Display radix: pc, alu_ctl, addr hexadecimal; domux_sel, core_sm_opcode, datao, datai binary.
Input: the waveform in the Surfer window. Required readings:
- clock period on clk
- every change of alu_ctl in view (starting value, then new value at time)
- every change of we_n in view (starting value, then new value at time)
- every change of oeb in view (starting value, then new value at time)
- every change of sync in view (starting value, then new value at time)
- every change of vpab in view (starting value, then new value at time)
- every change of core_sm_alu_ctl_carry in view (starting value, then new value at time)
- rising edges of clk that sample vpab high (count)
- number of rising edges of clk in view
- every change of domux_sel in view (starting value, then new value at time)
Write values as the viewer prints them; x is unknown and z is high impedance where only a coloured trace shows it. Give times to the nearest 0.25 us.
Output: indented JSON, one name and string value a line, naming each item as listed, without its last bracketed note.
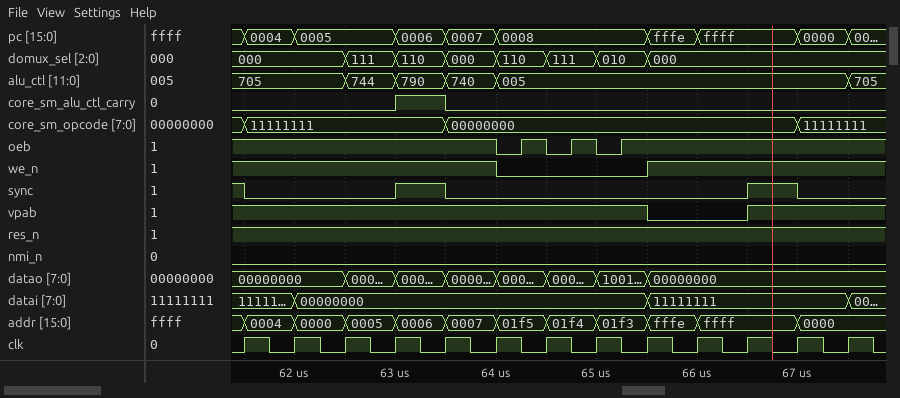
{
  "clock period on clk": "0.5 us",
  "every change of alu_ctl in view": "705, 744 at 62.5 us, 790 at 63 us, 740 at 63.5 us, 005 at 64 us, 705 at 67.5 us",
  "every change of we_n in view": "1, 0 at 64 us, 1 at 65.5 us",
  "every change of oeb in view": "1, 0 at 64 us, 1 at 64.25 us, 0 at 64.5 us, 1 at 64.75 us, 0 at 65 us, 1 at 65.25 us",
  "every change of sync in view": "1, 0 at 61.5 us, 1 at 63 us, 0 at 63.5 us, 1 at 66.5 us, 0 at 67 us",
  "every change of vpab in view": "1, 0 at 65.5 us, 1 at 66.5 us",
  "every change of core_sm_alu_ctl_carry in view": "0, 1 at 63 us, 0 at 63.5 us",
  "rising edges of clk that sample vpab high": "11",
  "number of rising edges of clk in view": "13",
  "every change of domux_sel in view": "000, 111 at 62.5 us, 110 at 63 us, 000 at 63.5 us, 110 at 64 us, 111 at 64.5 us, 010 at 65 us, 000 at 65.5 us"
}
